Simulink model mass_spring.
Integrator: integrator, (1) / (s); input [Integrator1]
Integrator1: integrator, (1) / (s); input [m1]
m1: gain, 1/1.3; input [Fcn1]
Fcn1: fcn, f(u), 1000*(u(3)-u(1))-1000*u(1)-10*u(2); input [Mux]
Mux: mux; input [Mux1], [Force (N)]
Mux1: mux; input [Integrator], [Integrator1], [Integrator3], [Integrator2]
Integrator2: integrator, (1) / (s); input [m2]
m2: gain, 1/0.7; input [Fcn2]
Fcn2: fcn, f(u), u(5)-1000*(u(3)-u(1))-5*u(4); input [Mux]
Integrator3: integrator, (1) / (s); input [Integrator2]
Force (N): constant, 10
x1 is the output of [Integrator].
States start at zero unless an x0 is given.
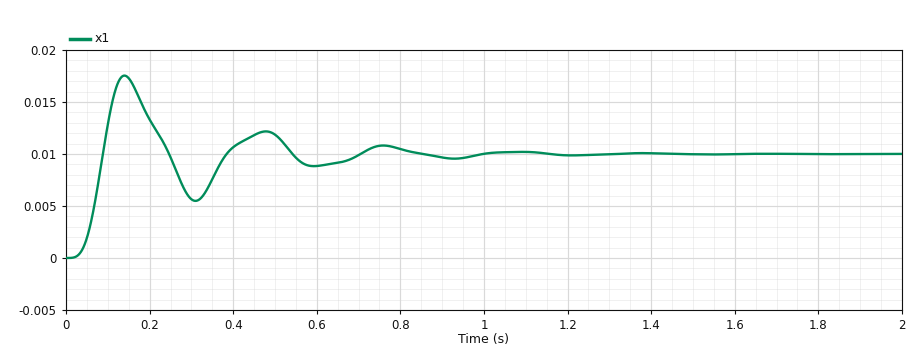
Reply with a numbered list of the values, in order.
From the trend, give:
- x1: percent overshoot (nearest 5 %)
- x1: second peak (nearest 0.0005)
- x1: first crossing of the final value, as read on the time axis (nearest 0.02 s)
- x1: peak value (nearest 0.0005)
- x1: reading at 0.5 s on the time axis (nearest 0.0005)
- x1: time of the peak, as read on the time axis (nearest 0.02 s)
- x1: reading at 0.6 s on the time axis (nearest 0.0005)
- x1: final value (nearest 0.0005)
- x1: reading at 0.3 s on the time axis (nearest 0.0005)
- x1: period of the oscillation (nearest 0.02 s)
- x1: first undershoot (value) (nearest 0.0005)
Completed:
1. 75 %
2. 0.0120
3. 0.08 s
4. 0.0175
5. 0.0120
6. 0.14 s
7. 0.0090
8. 0.0100
9. 0.0055
10. 0.34 s
11. 0.0055
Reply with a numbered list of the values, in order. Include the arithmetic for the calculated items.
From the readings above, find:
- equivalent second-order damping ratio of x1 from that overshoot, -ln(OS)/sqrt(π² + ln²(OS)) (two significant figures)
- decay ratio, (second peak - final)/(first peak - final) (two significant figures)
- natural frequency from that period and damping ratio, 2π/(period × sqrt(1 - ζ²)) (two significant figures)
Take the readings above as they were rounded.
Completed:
1. ln(0.75) = -0.288; 0.288 / sqrt(9.870 + 0.083) = 0.091
2. (0.012 - 0.01) / (0.0175 - 0.01) = 0.27
3. 2π / (0.34 × sqrt(1 - 0.091²)) = 19 rad/s
